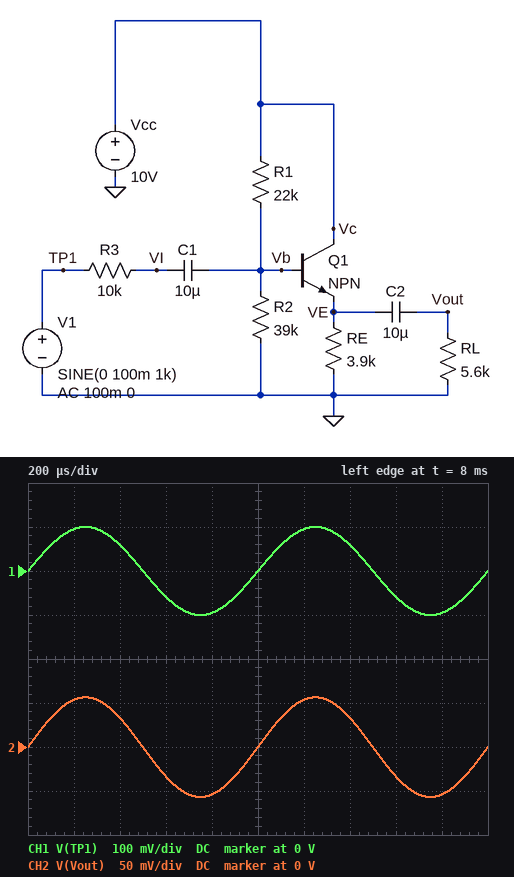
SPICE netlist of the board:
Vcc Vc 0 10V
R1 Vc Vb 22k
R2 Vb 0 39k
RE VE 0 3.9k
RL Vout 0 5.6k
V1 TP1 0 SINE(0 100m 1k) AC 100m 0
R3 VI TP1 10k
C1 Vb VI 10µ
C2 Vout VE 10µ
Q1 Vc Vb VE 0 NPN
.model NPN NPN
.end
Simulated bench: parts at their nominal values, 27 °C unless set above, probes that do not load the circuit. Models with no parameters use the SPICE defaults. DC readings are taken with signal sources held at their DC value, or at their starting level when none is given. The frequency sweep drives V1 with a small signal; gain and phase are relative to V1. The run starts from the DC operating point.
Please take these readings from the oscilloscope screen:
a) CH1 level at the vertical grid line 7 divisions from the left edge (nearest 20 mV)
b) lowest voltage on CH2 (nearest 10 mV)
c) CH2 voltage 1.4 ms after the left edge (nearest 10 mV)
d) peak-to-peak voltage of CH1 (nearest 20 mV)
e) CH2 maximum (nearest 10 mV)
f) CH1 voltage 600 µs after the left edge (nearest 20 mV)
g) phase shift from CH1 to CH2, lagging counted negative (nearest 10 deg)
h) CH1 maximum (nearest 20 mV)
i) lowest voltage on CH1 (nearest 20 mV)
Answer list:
60 mV
-60 mV
30 mV
200 mV
60 mV
-60 mV
0 deg
100 mV
-100 mV
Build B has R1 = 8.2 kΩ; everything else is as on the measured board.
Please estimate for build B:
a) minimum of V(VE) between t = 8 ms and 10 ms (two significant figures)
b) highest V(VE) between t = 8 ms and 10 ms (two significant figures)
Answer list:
7.3 V
7.4 V
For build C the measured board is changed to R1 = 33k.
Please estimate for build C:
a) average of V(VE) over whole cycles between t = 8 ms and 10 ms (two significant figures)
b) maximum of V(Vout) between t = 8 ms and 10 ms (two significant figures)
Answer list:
4.4 V
62 mV
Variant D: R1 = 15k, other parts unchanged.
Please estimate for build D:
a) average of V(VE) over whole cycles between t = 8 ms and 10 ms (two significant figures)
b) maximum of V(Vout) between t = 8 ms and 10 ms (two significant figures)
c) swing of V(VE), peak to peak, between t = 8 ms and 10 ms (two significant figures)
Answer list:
6.3 V
50 mV
100 mV
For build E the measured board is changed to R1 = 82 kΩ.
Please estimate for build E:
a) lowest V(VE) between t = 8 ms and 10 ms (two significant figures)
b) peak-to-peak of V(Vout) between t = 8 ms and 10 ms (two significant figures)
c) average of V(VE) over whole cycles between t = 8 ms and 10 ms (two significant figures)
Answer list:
2.2 V
140 mV
2.3 V
